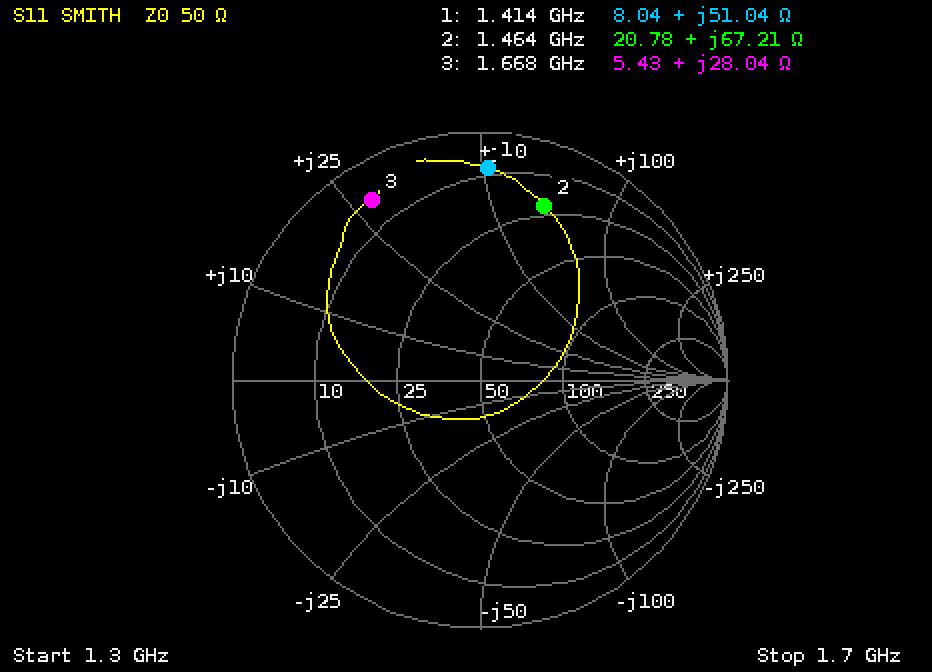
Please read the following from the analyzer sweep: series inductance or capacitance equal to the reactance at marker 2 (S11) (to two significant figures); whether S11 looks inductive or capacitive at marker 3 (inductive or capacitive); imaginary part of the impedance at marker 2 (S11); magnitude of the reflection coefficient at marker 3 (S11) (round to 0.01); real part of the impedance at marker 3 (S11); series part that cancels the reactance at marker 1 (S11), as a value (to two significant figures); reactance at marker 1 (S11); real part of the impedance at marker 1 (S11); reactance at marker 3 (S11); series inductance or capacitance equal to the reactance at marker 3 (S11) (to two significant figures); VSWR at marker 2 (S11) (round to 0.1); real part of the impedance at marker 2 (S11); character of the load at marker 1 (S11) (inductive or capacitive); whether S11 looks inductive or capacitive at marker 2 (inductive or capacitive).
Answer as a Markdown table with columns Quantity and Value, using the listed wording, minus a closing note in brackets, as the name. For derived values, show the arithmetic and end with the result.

| Quantity | Value |
|---|---|
| series inductance or capacitance equal to the reactance at marker 2 (S11) | L = 67.21 Ω/(2π × 1.464 GHz) ≈ 7.3 nH |
| whether S11 looks inductive or capacitive at marker 3 | inductive |
| imaginary part of the impedance at marker 2 | +67.21 Ω |
| magnitude of the reflection coefficient at marker 3 (S11) | 0.85 |
| real part of the impedance at marker 3 | 5.43 Ω |
| series part that cancels the reactance at marker 1 (S11), as a value | C = 1/(2π × 1.414 GHz × 51.04 Ω) ≈ 2.2 pF |
| reactance at marker 1 | +51.04 Ω |
| real part of the impedance at marker 1 | 8.04 Ω |
| reactance at marker 3 | +28.04 Ω |
| series inductance or capacitance equal to the reactance at marker 3 (S11) | L = 28.04 Ω/(2π × 1.668 GHz) ≈ 2.7 nH |
| VSWR at marker 2 (S11) | 7.0 |
| real part of the impedance at marker 2 | 20.78 Ω |
| character of the load at marker 1 (S11) | inductive |
| whether S11 looks inductive or capacitive at marker 2 | inductive |
